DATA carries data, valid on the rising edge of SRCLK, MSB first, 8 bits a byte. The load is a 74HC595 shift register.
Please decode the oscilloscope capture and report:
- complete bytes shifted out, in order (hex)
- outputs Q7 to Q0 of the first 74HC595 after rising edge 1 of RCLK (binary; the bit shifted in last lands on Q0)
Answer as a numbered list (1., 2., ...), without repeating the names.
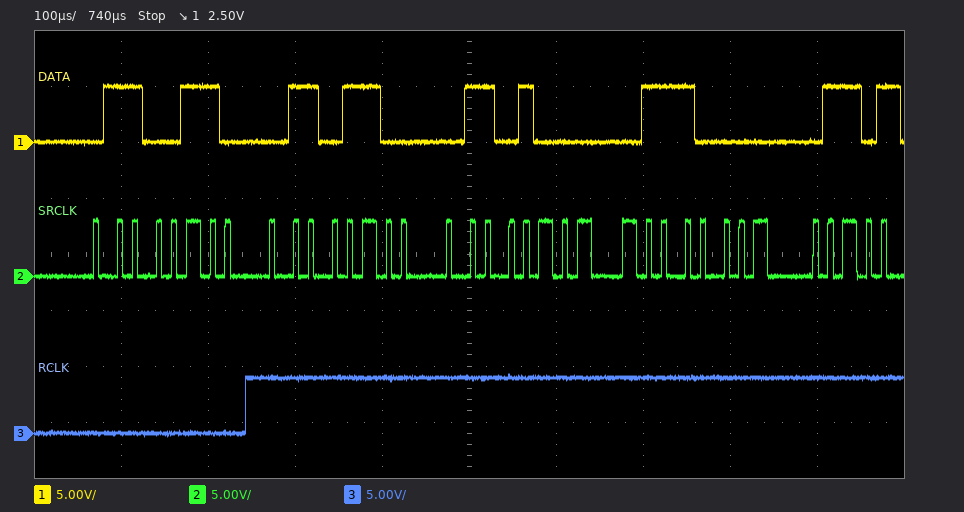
1. 0x66 0x6C 0x68 0x70
2. 01100110
